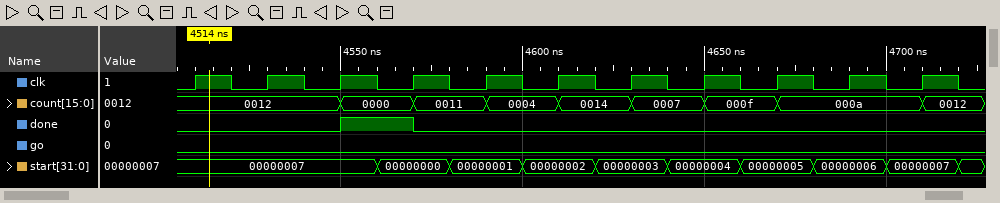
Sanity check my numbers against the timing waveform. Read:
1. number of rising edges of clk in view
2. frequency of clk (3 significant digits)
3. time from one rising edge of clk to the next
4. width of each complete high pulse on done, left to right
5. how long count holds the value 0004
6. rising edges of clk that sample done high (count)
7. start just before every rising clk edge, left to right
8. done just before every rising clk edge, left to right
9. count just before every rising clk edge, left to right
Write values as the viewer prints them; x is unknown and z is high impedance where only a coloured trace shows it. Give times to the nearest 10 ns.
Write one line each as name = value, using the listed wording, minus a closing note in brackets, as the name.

number of rising edges of clk in view = 11
frequency of clk = 50.0 MHz
time from one rising edge of clk to the next = 20 ns
width of each complete high pulse on done, left to right = 20 ns
how long count holds the value 0004 = 20 ns
rising edges of clk that sample done high = 1
start just before every rising clk edge, left to right = 00000007, 00000007, 00000007, 00000000, 00000001, 00000002, 00000003, 00000004, 00000005, 00000006, 00000007
done just before every rising clk edge, left to right = 0 0 0 1 0 0 0 0 0 0 0
count just before every rising clk edge, left to right = 0012, 0012, 0012, 0000, 0011, 0004, 0014, 0007, 000f, 000a, 000a
